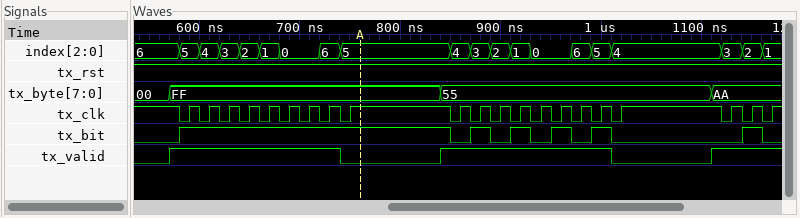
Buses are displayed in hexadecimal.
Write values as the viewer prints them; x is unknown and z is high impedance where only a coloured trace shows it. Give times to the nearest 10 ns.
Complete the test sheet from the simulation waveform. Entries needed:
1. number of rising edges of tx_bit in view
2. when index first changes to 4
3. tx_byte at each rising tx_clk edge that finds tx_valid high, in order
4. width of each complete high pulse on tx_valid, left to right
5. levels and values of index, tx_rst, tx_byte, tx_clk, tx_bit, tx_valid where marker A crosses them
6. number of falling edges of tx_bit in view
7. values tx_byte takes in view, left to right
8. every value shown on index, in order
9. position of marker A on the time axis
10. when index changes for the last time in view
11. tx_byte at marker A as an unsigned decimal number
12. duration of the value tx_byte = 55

6
600 ns
FF, FF, FF, FF, FF, FF, FF, FF, 55, 55, 55, 55, 55, 55, 55, 55, AA, AA, AA
170 ns, 170 ns
index=5, tx_rst=1, tx_byte=FF, tx_clk=1, tx_bit=1, tx_valid=0
6
00, FF, 55, AA
6, 5, 4, 3, 2, 1, 0, 6, 5, 4, 3, 2, 1, 0, 6, 5, 4, 3, 2, 1
760 ns
1160 ns
255
270 ns
